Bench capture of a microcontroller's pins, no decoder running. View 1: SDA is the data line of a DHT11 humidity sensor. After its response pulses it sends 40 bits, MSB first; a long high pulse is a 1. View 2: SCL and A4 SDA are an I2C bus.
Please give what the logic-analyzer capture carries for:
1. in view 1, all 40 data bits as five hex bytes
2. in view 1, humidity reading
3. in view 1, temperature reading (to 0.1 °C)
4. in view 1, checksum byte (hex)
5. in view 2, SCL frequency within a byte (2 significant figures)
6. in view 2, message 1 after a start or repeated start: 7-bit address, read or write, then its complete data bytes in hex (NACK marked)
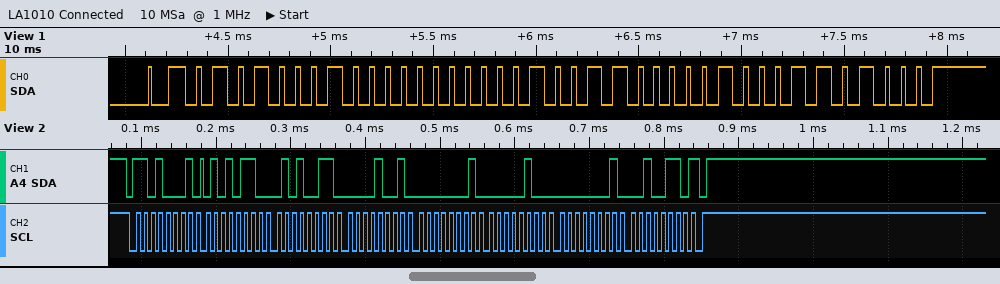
51 00 13 04 68
81 %
19.4 °C
0x68
100 kHz
0x68 read: 56 53 09 01 04 01 26 NACK
